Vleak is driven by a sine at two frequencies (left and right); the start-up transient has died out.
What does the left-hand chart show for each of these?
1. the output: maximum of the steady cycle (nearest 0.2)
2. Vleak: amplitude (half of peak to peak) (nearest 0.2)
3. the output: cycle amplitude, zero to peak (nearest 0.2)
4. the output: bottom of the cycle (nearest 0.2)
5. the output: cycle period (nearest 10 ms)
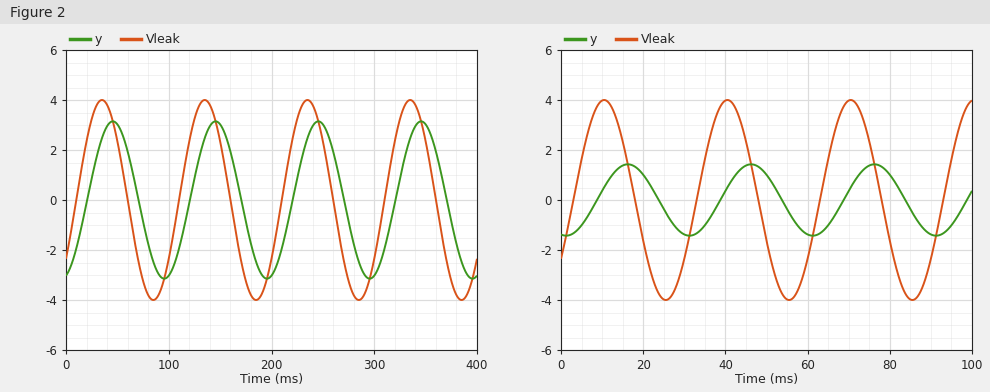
3.2
4.0
3.2
-3.2
100 ms
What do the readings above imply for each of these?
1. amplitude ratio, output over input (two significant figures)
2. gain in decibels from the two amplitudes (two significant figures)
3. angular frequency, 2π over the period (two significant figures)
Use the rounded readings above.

0.80
-1.9 dB
0.063 rad/ms
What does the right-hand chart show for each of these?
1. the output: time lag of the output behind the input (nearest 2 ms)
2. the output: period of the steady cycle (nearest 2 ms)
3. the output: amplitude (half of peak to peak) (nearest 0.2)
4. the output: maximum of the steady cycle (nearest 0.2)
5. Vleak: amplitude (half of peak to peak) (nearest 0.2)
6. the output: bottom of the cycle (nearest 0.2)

6 ms
30 ms
1.4
1.4
4.0
-1.4
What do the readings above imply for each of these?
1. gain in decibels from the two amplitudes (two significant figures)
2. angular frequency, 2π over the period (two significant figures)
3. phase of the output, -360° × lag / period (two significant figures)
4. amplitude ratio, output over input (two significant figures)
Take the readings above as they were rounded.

-9.1 dB
0.21 rad/ms
-72°
0.35
